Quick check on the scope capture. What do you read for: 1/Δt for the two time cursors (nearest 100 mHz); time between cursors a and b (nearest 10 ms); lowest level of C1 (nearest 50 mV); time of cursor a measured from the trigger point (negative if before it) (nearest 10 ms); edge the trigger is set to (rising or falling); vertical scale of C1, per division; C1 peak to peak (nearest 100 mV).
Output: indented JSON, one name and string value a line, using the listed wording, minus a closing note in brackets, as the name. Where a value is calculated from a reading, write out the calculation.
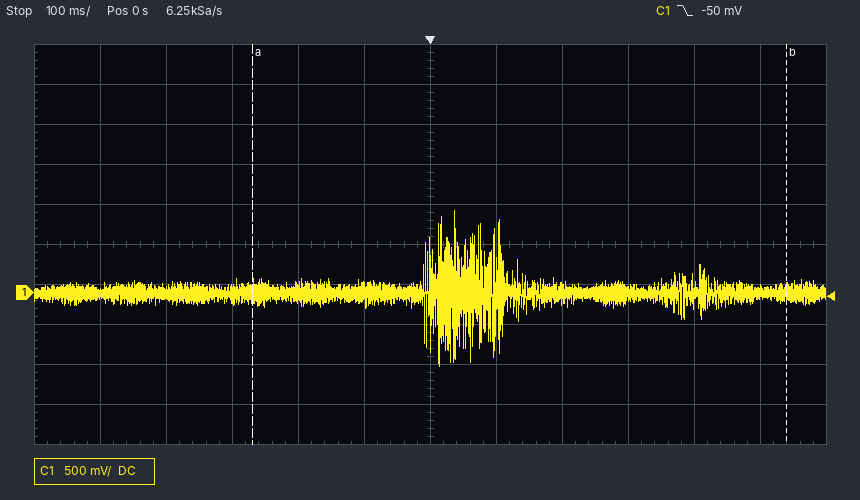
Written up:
{
  "1/Δt for the two time cursors": "1 / 810 ms ≈ 1.2 Hz",
  "time between cursors a and b": "810 ms",
  "lowest level of C1": "-900 mV",
  "time of cursor a measured from the trigger point (negative if before it)": "-270 ms",
  "edge the trigger is set to": "falling",
  "vertical scale of C1, per division": "500 mV",
  "C1 peak to peak": "1.90 V"
}
